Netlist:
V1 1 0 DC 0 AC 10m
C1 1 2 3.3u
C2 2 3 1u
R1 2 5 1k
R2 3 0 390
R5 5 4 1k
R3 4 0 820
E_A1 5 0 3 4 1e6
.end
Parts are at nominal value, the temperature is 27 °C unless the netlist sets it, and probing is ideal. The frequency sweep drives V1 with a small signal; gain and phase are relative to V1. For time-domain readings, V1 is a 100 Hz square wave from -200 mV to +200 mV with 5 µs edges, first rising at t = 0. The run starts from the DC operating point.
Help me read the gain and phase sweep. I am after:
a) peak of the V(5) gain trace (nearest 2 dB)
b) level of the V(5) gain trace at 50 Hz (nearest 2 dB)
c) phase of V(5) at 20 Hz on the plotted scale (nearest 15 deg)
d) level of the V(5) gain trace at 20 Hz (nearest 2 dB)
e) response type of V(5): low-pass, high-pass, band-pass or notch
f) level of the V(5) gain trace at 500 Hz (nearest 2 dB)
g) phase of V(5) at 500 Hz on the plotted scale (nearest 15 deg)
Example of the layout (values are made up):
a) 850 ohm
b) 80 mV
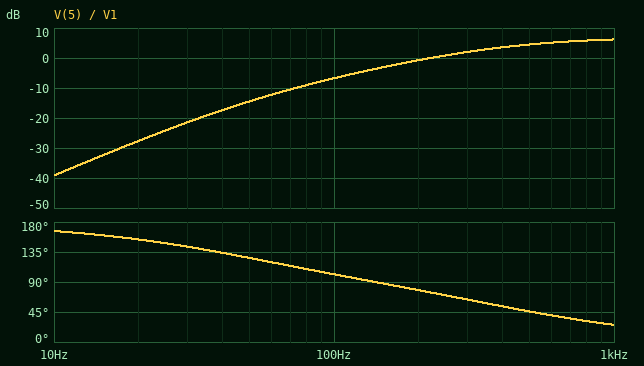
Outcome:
a) 6 dB
b) -14 dB
c) 150 deg
d) -28 dB
e) high-pass
f) 4 dB
g) 45 deg
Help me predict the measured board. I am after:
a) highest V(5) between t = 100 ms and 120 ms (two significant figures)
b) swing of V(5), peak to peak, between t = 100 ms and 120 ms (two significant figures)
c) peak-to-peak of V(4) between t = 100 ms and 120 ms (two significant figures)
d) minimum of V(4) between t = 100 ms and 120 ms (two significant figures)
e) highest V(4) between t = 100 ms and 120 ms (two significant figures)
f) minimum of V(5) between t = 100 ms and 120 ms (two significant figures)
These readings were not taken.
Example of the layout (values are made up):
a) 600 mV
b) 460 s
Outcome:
a) 900 mV
b) 1.8 V
c) 810 mV
d) -410 mV
e) 410 mV
f) -900 mV
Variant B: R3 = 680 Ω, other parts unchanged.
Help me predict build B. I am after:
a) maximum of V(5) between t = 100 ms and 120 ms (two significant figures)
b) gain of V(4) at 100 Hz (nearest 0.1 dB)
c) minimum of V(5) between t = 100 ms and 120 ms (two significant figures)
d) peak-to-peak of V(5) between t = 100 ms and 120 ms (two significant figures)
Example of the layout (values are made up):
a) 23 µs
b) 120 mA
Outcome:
a) 1.0 V
b) -13.5 dB
c) -1.0 V
d) 2.0 V
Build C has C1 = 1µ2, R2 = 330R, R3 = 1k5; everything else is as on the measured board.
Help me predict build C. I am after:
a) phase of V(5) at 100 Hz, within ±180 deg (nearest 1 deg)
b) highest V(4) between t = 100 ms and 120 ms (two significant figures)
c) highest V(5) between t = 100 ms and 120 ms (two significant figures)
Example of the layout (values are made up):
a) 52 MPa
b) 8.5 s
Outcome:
a) 124 deg
b) 400 mV
c) 660 mV
